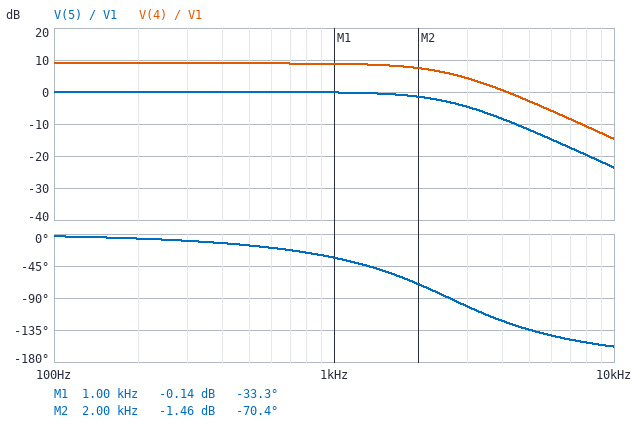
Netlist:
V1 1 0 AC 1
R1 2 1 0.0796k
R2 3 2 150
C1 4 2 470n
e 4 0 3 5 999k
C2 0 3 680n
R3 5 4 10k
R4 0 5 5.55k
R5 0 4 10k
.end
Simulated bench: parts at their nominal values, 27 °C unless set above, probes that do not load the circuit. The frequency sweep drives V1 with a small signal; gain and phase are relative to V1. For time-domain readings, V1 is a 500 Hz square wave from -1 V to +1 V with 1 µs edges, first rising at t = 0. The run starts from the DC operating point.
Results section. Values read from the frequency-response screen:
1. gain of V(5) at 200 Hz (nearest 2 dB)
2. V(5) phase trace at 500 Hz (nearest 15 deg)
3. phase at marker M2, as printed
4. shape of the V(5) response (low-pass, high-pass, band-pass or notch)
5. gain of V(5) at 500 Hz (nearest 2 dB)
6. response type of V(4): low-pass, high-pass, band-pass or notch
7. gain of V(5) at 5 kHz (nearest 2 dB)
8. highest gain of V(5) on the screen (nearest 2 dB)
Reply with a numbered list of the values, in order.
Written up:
1. 0 dB
2. -15 deg
3. -70.4 deg
4. low-pass
5. 0 dB
6. low-pass
7. -12 dB
8. 0 dB
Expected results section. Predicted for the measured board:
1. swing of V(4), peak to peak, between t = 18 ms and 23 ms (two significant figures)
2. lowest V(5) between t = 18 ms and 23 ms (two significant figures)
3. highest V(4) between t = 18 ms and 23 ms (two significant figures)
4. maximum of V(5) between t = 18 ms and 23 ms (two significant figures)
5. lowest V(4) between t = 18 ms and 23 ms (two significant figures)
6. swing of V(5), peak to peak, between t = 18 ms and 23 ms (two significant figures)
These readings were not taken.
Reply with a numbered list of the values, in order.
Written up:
1. 6.0 V
2. -1.1 V
3. 3.0 V
4. 1.1 V
5. -3.0 V
6. 2.2 V
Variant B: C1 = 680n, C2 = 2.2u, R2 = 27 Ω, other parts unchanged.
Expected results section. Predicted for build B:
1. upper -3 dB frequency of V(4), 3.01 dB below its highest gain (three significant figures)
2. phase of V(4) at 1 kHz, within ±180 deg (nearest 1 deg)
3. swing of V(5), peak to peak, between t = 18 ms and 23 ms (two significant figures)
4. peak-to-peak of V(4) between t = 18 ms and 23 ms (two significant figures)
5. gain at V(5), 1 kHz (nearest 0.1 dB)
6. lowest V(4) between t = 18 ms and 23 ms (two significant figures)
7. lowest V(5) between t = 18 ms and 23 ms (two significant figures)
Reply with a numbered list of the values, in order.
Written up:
1. 1.39 kHz
2. -45 deg
3. 2.0 V
4. 5.6 V
5. -1.8 dB
6. -2.8 V
7. -1.0 V
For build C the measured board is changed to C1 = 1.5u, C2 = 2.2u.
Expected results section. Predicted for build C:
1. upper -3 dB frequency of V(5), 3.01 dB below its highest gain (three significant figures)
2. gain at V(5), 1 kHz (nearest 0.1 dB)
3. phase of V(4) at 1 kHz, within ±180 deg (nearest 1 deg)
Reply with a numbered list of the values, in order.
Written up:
1. 775 Hz
2. -5.6 dB
3. -107 deg
